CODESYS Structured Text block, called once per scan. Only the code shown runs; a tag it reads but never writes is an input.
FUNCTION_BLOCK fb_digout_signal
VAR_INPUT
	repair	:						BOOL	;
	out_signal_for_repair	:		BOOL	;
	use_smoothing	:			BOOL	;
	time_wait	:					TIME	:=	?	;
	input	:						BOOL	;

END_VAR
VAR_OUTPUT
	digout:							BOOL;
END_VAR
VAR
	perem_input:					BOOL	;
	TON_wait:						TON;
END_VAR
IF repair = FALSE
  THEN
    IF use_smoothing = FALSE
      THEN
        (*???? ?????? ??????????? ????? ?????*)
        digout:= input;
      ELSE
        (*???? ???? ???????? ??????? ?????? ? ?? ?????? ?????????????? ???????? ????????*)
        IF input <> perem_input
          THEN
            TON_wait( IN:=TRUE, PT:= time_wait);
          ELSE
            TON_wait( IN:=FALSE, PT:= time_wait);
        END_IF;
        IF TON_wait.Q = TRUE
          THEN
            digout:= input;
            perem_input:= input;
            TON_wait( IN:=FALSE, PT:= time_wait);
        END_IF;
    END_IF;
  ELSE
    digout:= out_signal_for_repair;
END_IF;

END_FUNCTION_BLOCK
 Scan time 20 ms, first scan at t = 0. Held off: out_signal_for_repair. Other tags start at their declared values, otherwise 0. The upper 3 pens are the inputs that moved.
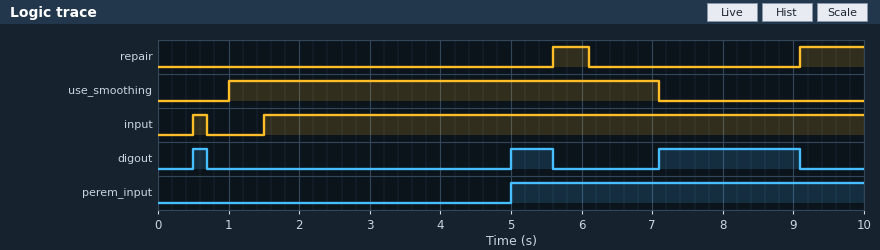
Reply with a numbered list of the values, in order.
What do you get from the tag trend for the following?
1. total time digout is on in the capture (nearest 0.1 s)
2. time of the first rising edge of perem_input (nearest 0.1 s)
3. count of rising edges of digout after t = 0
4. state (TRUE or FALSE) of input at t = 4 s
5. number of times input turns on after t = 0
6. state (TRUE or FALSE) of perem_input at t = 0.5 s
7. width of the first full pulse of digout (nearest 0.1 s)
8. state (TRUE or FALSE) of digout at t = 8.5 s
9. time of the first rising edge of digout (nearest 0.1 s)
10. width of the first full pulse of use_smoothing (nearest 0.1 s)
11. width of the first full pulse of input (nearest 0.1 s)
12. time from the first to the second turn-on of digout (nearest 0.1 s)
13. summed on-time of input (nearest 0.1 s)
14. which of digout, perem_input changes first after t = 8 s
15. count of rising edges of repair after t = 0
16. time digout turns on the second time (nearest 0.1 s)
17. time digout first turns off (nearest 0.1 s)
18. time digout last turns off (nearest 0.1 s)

1. 2.8 s
2. 5.0 s
3. 3
4. TRUE
5. 2
6. FALSE
7. 0.2 s
8. TRUE
9. 0.5 s
10. 6.1 s
11. 0.2 s
12. 4.5 s
13. 8.7 s
14. digout
15. 2
16. 5.0 s
17. 0.7 s
18. 9.1 s
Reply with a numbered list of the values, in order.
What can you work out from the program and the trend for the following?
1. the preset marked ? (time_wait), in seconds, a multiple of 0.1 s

1. 3.5 s
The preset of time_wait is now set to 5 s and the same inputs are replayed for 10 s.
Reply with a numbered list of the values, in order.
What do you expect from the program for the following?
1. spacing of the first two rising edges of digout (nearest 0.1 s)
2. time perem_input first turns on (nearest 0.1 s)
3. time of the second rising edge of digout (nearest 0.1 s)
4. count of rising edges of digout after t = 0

1. 6.0 s
2. 6.5 s
3. 6.5 s
4. 2
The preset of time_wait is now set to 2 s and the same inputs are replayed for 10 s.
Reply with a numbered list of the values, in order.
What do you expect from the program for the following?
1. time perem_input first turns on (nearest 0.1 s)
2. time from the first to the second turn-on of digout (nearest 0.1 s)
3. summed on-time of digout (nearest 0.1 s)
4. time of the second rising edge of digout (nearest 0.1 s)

1. 3.5 s
2. 3.0 s
3. 4.3 s
4. 3.5 s
